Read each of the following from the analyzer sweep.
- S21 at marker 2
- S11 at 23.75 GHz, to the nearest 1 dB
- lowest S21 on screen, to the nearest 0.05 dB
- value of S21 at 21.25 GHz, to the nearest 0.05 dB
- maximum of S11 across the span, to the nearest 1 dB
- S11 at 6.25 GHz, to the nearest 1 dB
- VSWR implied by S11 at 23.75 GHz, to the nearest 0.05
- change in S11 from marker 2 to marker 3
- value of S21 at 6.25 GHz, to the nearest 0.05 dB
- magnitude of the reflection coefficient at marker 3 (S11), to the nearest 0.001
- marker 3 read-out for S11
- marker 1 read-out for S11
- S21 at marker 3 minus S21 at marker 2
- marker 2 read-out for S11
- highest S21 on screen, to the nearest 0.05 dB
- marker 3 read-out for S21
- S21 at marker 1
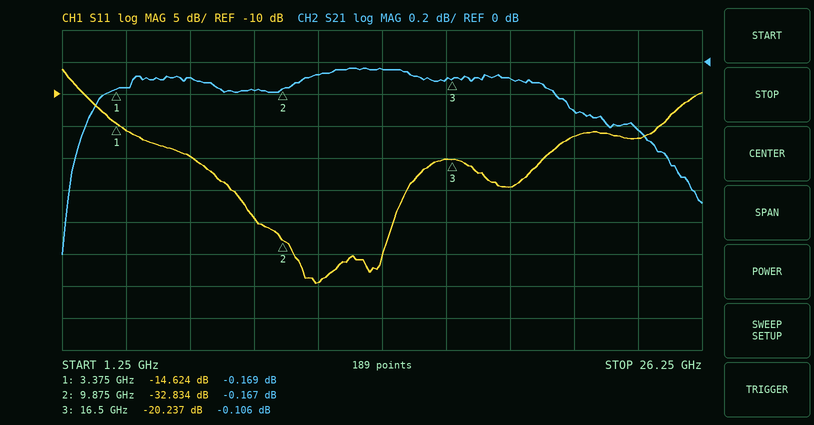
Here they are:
-0.167 dB
-17 dB
-1.20 dB
-0.30 dB
-6 dB
-20 dB
1.35
12.597 dB
-0.10 dB
0.097
-20.237 dB
-14.624 dB
0.061 dB
-32.834 dB
-0.05 dB
-0.106 dB
-0.169 dB
